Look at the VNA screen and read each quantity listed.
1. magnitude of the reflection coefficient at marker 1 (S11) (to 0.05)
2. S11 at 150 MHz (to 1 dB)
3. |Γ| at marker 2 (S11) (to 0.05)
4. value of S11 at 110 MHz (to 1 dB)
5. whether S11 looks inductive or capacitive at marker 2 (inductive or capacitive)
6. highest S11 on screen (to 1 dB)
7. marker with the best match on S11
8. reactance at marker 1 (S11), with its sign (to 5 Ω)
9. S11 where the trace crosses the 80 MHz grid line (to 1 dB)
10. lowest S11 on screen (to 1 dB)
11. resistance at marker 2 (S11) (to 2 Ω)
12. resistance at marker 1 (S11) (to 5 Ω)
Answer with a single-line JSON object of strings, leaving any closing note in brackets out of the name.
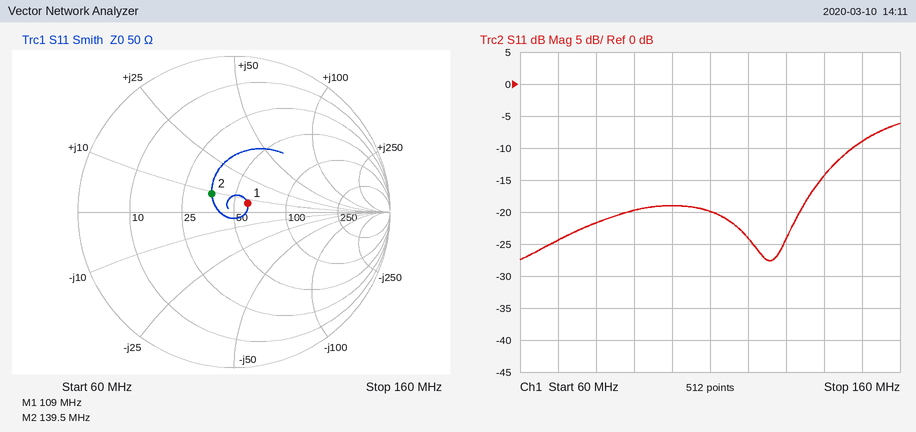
{"magnitude of the reflection coefficient at marker 1 (S11)": "0.10", "S11 at 150 MHz": "-9 dB", "|Γ| at marker 2 (S11)": "0.20", "value of S11 at 110 MHz": "-20 dB", "whether S11 looks inductive or capacitive at marker 2": "inductive", "highest S11 on screen": "-6 dB", "marker with the best match on S11": "marker 1", "reactance at marker 1 (S11), with its sign": "+5 Ω", "S11 where the trace crosses the 80 MHz grid line": "-22 dB", "lowest S11 on screen": "-28 dB", "resistance at marker 2 (S11)": "36 Ω", "resistance at marker 1 (S11)": "60 Ω"}
